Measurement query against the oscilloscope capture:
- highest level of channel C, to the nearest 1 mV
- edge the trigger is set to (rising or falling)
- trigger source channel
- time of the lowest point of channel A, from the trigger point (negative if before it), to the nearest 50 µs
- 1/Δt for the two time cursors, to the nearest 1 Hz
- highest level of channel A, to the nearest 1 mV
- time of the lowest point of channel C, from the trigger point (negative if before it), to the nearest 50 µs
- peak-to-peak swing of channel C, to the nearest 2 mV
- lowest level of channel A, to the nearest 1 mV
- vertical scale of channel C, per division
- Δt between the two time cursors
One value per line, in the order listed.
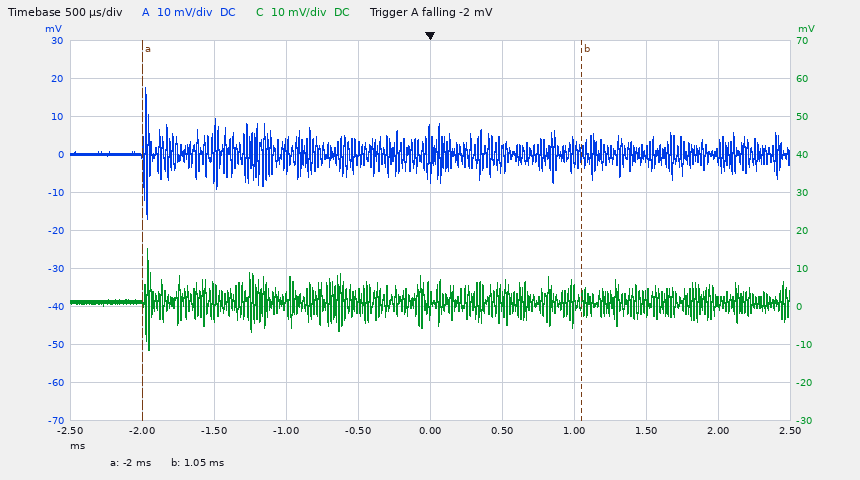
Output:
15 mV
falling
channel A
-1.95 ms
328 Hz
18 mV
-1.95 ms
26 mV
-17 mV
10 mV
3.05 ms
